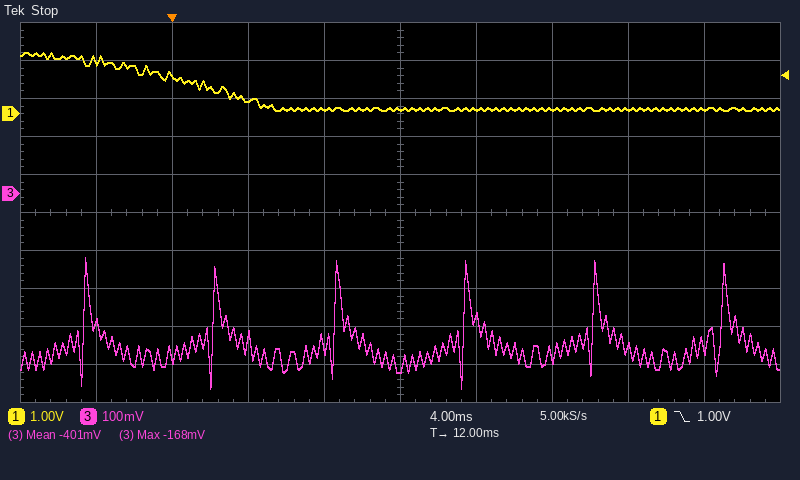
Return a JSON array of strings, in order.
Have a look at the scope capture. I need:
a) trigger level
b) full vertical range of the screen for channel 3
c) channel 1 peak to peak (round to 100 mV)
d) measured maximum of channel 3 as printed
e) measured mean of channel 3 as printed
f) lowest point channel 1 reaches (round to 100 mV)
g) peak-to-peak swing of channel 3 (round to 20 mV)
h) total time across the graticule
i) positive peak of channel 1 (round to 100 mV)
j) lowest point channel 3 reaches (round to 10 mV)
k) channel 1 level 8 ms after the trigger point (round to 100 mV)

["1.00 V", "1 V", "1.5 V", "-168 mV", "-401 mV", "100 mV", "340 mV", "40 ms", "1.6 V", "-510 mV", "100 mV"]
